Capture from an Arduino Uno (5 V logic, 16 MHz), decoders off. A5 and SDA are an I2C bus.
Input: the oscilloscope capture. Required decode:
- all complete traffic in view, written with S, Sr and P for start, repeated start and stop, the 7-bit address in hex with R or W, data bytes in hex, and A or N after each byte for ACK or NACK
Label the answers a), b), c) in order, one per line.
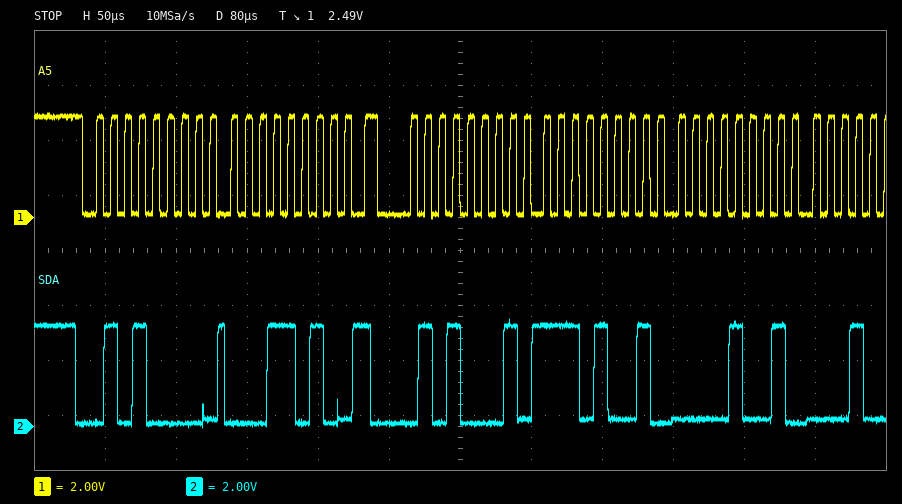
a) S 28W A 1A A Sr 28R A E9 A 09 A
